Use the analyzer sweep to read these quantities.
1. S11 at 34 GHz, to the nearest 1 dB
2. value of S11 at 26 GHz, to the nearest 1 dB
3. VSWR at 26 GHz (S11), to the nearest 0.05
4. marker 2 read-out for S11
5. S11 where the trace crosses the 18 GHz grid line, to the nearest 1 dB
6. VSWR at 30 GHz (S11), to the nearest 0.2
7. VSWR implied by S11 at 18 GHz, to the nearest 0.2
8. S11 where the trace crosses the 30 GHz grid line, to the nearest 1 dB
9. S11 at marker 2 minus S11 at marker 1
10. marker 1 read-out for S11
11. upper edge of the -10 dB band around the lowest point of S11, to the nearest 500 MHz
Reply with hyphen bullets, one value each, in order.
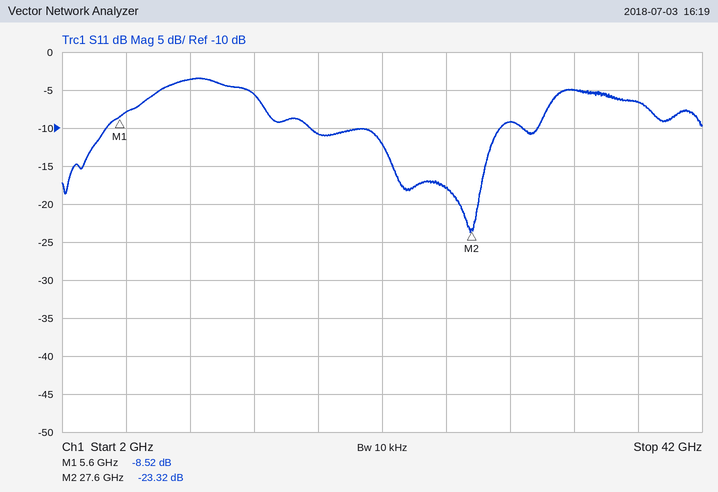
- -5 dB
- -18 dB
- 1.30
- -23.32 dB
- -11 dB
- 2.0
- 1.8
- -9 dB
- -14.80 dB
- -8.52 dB
- 29.5 GHz
